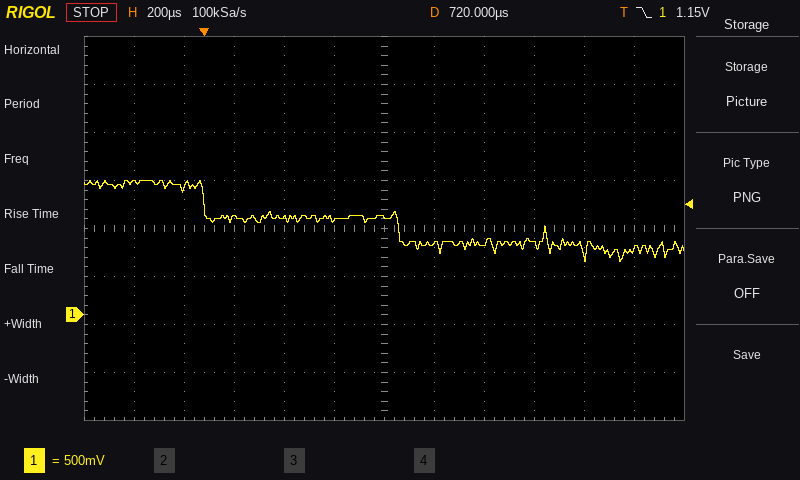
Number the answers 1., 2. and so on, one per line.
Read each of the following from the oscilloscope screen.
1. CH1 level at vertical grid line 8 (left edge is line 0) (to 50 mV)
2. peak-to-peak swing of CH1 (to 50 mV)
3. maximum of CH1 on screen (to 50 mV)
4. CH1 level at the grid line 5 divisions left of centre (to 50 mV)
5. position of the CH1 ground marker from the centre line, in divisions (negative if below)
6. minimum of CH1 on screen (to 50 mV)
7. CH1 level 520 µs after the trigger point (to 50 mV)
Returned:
1. 750 mV
2. 850 mV
3. 1.40 V
4. 1.40 V
5. -1.8 div
6. 550 mV
7. 1.00 V
